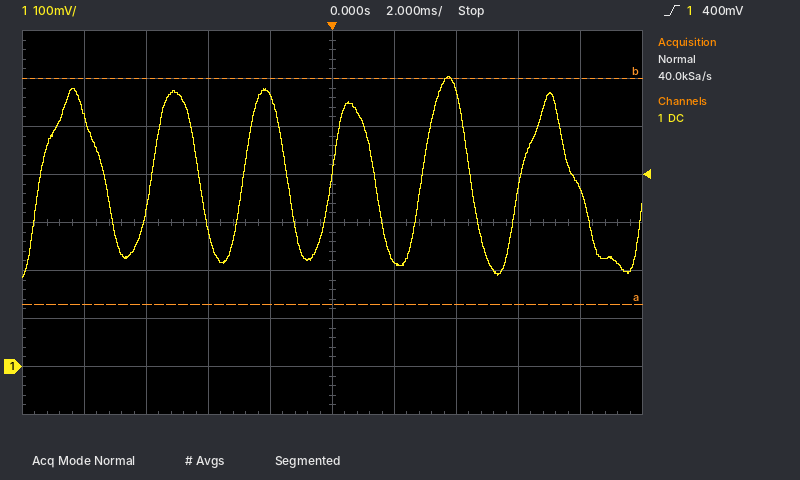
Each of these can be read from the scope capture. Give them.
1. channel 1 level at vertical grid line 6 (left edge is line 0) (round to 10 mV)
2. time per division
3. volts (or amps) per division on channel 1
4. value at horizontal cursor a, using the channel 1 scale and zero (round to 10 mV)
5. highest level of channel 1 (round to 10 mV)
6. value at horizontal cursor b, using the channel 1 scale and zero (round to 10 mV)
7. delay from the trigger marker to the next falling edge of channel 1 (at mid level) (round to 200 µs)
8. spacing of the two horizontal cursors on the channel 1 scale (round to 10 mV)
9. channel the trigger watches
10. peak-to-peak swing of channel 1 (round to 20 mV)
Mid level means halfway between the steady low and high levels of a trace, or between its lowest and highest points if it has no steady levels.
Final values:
220 mV
2 ms
100 mV
130 mV
600 mV
600 mV
1.4 ms
470 mV
channel 1
420 mV
